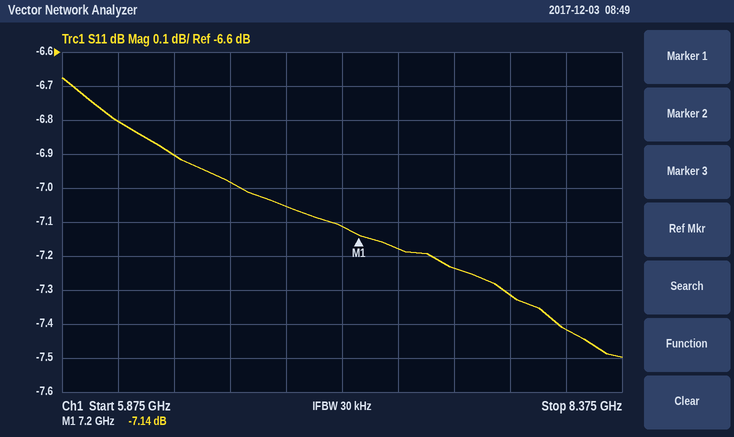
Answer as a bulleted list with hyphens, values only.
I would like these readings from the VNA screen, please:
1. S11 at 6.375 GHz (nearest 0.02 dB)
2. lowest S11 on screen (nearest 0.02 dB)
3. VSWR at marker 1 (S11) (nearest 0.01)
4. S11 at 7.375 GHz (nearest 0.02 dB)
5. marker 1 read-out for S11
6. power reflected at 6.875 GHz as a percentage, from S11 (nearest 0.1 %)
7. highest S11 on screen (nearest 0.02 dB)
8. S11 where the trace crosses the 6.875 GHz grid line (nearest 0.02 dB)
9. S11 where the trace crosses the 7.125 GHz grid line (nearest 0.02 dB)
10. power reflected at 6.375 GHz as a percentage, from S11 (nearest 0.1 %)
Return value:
- -6.90 dB
- -7.50 dB
- 2.57
- -7.18 dB
- -7.14 dB
- 19.7 %
- -6.68 dB
- -7.06 dB
- -7.12 dB
- 20.4 %
